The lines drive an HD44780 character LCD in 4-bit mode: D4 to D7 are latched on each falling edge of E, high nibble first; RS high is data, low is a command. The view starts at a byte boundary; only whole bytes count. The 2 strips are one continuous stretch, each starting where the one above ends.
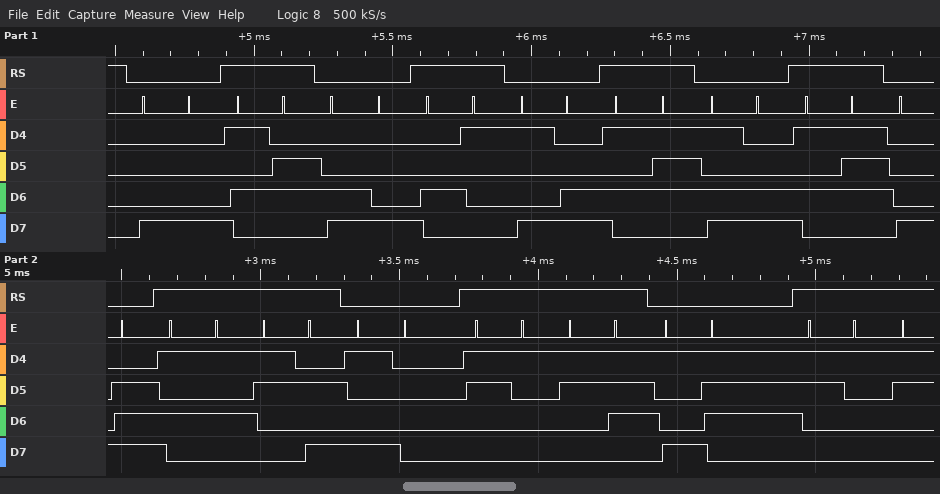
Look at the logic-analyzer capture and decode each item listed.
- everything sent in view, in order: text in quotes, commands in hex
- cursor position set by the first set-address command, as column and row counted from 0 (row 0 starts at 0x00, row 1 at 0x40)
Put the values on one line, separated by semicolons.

0x88 "V" 0xC8 "A" 0x9C "W" 0xDC "W" 0x8E "U:" 0x90 "17" 0x97 "1"; column 8, row 0
